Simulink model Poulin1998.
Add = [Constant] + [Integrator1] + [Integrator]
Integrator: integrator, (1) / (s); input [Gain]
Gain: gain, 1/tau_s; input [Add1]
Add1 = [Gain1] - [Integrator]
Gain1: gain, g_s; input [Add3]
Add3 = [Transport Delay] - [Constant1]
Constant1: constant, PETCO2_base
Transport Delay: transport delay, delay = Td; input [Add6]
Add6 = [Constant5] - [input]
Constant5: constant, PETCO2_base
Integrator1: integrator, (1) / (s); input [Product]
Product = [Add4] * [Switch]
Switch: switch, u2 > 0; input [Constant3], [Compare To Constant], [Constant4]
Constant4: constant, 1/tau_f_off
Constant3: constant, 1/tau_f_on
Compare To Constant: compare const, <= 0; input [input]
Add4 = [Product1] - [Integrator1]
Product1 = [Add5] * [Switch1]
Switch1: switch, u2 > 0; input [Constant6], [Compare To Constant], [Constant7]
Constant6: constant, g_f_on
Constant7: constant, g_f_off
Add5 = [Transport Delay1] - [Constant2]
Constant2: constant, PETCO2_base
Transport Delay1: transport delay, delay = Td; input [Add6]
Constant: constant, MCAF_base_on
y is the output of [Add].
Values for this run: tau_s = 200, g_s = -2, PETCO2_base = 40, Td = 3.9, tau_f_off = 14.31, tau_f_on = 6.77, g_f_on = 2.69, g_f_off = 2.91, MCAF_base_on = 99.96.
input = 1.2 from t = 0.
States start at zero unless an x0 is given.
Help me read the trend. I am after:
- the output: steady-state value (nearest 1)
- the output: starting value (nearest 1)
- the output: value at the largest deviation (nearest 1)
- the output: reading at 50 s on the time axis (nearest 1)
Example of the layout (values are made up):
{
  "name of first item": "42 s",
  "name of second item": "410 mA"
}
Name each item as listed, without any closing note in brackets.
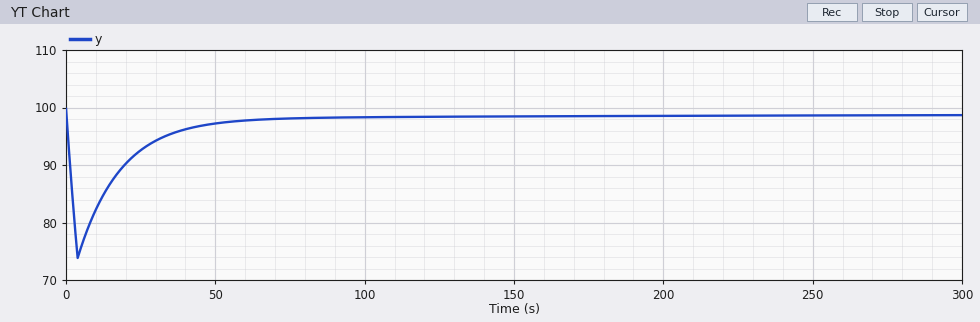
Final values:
{
  "the output: steady-state value": "99",
  "the output: starting value": "100",
  "the output: value at the largest deviation": "74",
  "the output: reading at 50 s on the time axis": "97"
}
